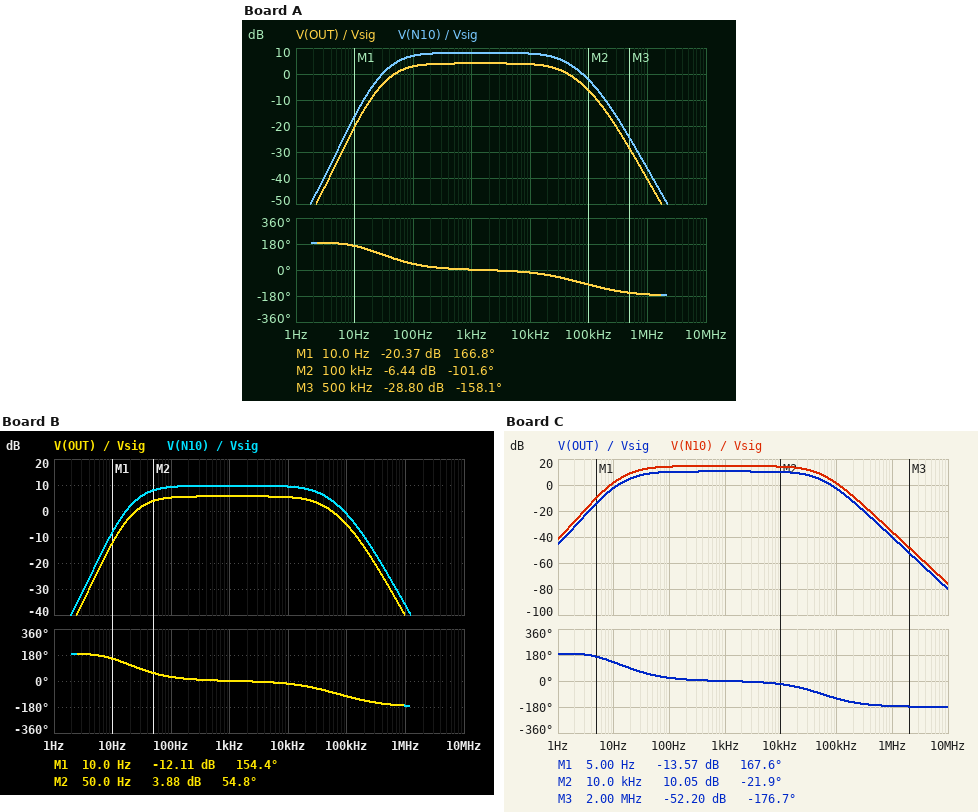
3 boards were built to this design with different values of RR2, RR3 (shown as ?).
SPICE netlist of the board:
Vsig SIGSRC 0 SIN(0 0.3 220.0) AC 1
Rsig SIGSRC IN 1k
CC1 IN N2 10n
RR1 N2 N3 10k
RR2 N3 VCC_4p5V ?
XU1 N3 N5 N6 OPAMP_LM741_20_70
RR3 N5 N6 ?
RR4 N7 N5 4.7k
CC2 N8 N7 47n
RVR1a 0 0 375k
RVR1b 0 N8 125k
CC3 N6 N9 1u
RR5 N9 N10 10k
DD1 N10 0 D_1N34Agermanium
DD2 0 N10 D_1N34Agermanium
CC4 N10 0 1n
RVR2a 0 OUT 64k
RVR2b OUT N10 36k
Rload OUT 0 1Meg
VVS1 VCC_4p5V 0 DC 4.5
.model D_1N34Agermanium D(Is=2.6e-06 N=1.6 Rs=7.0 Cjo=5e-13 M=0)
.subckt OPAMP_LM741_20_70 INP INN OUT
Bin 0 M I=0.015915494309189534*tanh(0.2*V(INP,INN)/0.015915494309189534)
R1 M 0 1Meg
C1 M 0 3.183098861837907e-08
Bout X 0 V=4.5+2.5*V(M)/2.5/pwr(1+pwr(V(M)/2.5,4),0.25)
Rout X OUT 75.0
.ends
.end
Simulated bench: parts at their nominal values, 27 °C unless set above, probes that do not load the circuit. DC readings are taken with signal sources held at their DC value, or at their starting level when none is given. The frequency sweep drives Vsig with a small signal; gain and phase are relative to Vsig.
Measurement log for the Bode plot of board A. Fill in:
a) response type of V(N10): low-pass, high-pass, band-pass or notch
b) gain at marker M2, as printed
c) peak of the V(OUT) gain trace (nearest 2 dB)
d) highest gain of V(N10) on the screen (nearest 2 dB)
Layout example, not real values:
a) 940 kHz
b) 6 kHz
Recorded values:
a) band-pass
b) -6.44 dB
c) 4 dB
d) 8 dB
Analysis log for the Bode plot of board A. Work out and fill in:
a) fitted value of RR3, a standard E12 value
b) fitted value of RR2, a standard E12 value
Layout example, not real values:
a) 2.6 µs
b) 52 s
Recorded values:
a) 680 kΩ
b) 330 kΩ
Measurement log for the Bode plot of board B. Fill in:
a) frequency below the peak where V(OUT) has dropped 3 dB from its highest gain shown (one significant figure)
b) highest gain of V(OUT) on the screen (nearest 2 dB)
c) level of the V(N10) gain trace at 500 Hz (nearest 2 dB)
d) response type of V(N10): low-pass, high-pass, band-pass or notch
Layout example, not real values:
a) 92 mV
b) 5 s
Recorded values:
a) 40 Hz
b) 6 dB
c) 10 dB
d) band-pass
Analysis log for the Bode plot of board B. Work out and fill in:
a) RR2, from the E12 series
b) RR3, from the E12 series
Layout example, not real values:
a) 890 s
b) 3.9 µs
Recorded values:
a) 820 kΩ
b) 820 kΩ
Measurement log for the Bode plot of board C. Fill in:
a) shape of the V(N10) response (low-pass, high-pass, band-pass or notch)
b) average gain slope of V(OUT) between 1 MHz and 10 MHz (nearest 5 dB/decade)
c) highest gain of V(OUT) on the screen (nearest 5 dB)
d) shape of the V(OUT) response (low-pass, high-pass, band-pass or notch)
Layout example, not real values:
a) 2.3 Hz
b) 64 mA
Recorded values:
a) band-pass
b) -40 dB/decade
c) 10 dB
d) band-pass
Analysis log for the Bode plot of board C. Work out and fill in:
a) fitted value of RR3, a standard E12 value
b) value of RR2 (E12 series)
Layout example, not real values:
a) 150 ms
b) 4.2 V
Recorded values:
a) 1.5 MΩ
b) 2.7 MΩ
